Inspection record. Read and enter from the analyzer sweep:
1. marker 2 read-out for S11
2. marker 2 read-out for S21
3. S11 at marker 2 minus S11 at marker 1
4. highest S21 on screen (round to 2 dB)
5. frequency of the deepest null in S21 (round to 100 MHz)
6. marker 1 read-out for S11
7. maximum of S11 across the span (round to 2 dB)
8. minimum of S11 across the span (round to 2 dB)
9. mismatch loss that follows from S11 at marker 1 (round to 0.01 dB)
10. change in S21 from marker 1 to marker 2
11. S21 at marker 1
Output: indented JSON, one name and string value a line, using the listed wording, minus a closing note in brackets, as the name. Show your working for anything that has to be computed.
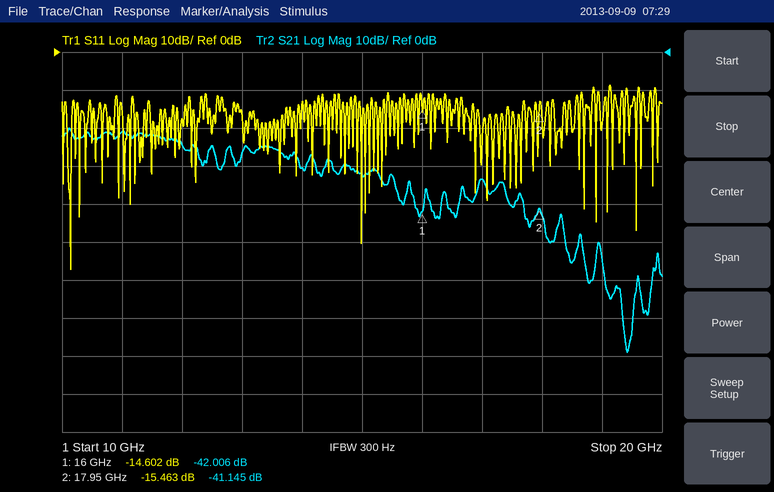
{
  "marker 2 read-out for S11": "-15.463 dB",
  "marker 2 read-out for S21": "-41.145 dB",
  "S11 at marker 2 minus S11 at marker 1": "-15.463 − (-14.602) = -0.861 dB",
  "highest S21 on screen": "-20 dB",
  "frequency of the deepest null in S21": "19.4 GHz",
  "marker 1 read-out for S11": "-14.602 dB",
  "maximum of S11 across the span": "-8 dB",
  "minimum of S11 across the span": "-58 dB",
  "mismatch loss that follows from S11 at marker 1": "−10 log10(1 − 10^(-14.602/10)) ≈ 0.15 dB",
  "change in S21 from marker 1 to marker 2": "-41.145 − (-42.006) = 0.861 dB",
  "S21 at marker 1": "-42.006 dB"
}
